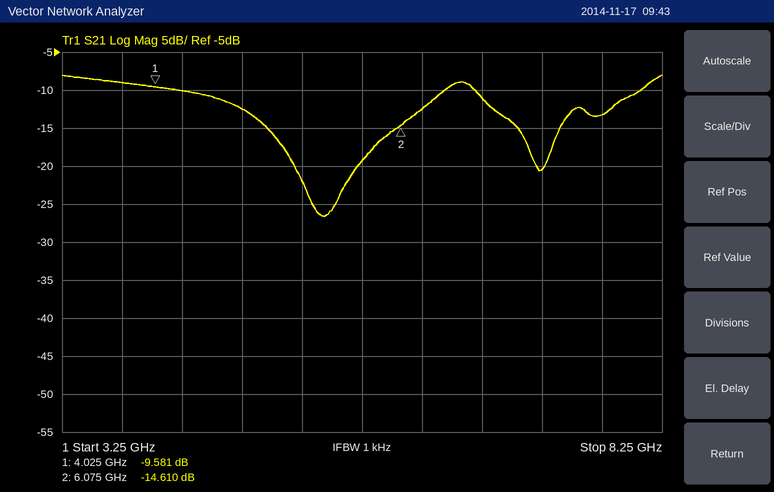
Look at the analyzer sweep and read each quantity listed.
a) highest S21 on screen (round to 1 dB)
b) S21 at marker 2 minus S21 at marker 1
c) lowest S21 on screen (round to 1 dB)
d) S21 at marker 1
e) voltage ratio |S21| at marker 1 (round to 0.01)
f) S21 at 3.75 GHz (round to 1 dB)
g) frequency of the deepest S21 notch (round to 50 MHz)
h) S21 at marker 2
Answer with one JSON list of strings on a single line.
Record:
["-8 dB", "-5.029 dB", "-27 dB", "-9.581 dB", "0.33", "-9 dB", "5.45 GHz", "-14.610 dB"]
